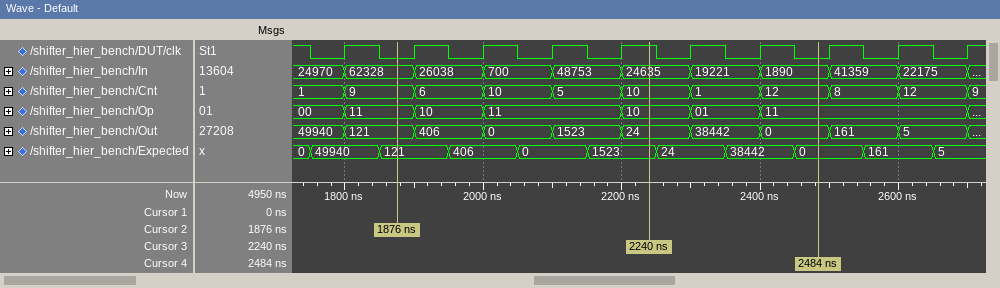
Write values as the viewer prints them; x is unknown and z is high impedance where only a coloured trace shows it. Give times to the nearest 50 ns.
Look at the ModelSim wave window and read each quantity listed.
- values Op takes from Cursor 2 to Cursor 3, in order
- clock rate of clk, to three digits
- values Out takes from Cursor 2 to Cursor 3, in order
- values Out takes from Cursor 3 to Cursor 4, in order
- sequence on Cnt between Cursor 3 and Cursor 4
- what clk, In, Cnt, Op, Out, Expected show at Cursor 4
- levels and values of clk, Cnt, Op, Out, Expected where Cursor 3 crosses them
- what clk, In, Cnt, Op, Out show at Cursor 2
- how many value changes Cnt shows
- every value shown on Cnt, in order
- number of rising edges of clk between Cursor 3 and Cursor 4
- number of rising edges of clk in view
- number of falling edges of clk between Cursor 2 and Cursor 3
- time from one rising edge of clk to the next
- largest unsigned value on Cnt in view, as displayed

11, 10, 11, 10
10.0 MHz
121, 406, 0, 1523, 24
24, 38442, 0
10, 1, 12
clk=0, In=1890, Cnt=12, Op=11, Out=0, Expected=0
clk=1, Cnt=10, Op=10, Out=24, Expected=1523
clk=0, In=62328, Cnt=9, Op=11, Out=121
10
1, 9, 6, 10, 5, 10, 1, 12, 8, 12, 9
2
10
3
100 ns
12
